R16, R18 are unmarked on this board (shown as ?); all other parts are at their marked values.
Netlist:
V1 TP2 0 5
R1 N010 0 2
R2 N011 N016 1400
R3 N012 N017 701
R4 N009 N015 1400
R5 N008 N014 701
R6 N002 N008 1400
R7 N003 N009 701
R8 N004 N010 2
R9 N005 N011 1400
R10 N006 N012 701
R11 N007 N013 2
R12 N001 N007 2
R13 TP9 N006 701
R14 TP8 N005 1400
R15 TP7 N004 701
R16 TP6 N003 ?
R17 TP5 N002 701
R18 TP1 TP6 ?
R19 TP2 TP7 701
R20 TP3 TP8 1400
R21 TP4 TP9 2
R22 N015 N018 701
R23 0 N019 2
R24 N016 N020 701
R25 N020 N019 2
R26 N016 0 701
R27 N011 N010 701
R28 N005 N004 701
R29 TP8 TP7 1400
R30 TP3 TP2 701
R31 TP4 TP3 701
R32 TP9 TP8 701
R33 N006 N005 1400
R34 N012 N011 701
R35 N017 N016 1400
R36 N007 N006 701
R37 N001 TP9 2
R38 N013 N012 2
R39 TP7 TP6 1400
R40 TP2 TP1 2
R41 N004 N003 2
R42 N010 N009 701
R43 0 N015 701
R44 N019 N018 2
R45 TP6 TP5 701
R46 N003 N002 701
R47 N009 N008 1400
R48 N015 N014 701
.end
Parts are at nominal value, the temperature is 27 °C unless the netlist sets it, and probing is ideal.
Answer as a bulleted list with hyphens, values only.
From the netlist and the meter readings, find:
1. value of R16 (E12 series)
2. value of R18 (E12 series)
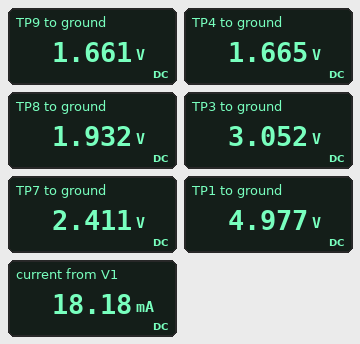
- 220 Ω
- 220 Ω
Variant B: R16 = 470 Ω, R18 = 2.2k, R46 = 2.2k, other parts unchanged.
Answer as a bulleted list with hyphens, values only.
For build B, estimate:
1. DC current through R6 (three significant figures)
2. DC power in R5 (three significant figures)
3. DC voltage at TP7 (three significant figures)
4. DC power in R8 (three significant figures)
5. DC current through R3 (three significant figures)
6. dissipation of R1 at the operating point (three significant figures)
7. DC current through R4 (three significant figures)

- 206 µA
- 8.12 µW
- 2.16 V
- 86.7 µW
- 609 µA
- 117 µW
- 9.70 µA
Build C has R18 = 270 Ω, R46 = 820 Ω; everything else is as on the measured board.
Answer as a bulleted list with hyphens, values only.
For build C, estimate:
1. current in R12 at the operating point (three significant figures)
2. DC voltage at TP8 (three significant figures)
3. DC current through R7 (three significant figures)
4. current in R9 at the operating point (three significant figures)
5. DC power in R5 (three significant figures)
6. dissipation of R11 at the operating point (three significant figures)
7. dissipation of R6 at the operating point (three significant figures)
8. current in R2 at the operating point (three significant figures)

- 2.19 mA
- 1.92 V
- 21.0 µA
- 79.5 µA
- 17.7 µW
- 8.23 µW
- 122 µW
- 306 µA
